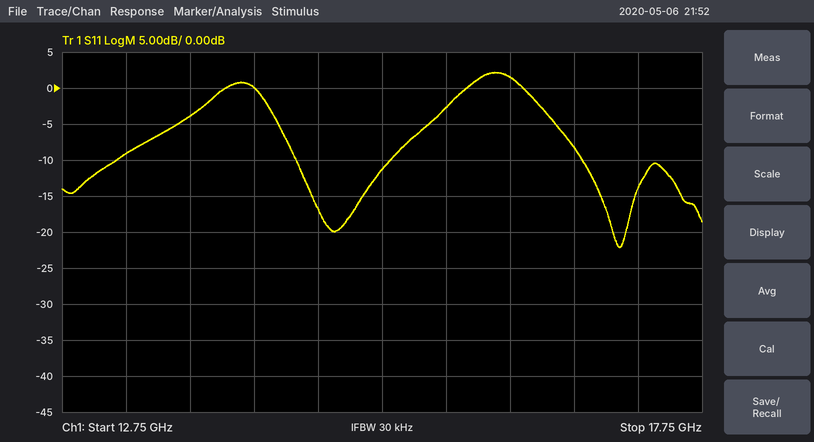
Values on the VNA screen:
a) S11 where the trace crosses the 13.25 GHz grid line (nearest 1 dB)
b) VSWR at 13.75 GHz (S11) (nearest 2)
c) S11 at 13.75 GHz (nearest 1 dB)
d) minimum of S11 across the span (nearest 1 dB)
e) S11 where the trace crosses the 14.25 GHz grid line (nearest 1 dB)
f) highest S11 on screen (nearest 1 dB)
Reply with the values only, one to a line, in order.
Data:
-9 dB
4
-4 dB
-22 dB
0 dB
2 dB
